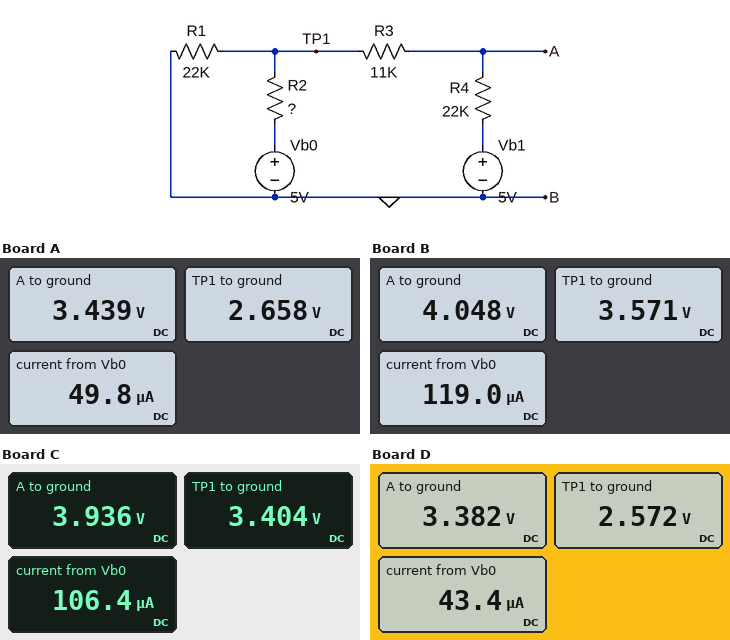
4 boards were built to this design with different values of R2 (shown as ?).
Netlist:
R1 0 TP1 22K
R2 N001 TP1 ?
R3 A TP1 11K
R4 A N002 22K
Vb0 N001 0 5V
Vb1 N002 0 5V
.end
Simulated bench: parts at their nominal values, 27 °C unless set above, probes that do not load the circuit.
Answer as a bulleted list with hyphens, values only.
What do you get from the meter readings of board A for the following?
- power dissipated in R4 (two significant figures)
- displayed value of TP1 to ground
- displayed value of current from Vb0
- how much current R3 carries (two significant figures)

- 110 µW
- 2.658 V
- 49.8 µA
- 71 µA
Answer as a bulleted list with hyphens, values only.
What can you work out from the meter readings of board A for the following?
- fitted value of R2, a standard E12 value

- 47 kΩ
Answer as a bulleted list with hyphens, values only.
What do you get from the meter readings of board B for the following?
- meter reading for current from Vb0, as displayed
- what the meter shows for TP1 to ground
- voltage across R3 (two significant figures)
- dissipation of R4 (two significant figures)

- 119.0 µA
- 3.571 V
- 480 mV
- 41 µW
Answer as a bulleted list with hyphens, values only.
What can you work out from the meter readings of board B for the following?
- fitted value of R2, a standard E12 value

- 12 kΩ
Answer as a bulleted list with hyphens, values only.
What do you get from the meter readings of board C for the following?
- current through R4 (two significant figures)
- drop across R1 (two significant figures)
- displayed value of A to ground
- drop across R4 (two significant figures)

- 48 µA
- 3.4 V
- 3.936 V
- 1.1 V
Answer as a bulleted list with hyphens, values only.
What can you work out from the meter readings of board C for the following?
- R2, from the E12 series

- 15 kΩ
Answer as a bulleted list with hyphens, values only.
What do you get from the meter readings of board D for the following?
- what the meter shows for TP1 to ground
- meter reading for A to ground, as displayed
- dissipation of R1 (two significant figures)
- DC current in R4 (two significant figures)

- 2.572 V
- 3.382 V
- 300 µW
- 74 µA
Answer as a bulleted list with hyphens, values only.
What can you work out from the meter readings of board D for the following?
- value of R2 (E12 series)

- 56 kΩ
